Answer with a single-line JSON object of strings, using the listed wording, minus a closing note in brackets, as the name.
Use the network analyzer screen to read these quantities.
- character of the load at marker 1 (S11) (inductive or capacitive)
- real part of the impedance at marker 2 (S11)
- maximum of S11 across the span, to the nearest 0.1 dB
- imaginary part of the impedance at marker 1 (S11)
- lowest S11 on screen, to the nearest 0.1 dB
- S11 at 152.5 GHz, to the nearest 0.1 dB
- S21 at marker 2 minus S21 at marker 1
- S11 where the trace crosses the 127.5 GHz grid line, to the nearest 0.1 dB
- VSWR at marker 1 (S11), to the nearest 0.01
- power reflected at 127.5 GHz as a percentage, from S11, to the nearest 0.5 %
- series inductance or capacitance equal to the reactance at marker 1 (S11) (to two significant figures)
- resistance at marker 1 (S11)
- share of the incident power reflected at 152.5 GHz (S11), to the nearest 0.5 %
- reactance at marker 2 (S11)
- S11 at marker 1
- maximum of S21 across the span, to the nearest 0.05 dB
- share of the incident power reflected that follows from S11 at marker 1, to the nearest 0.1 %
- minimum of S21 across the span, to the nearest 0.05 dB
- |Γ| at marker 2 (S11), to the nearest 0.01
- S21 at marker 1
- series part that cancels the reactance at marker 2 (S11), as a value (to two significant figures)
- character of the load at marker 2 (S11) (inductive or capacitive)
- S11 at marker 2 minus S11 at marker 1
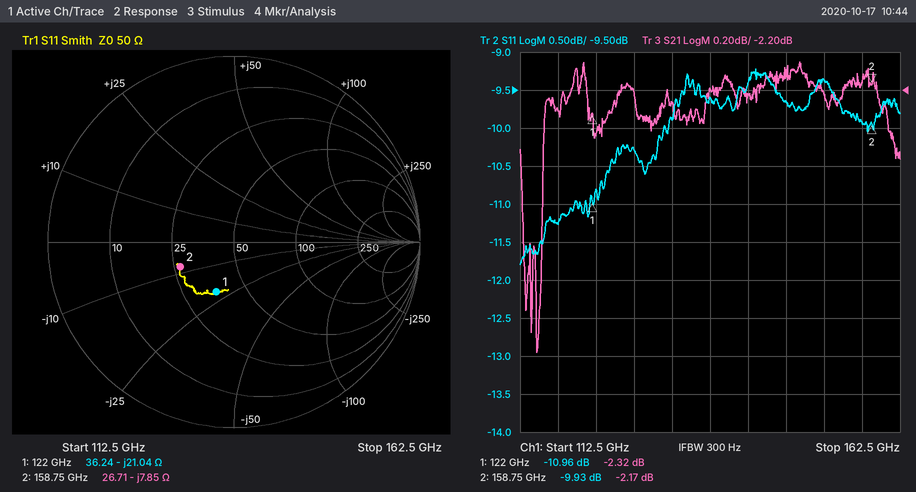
{"character of the load at marker 1 (S11)": "capacitive", "real part of the impedance at marker 2": "26.71 Ω", "maximum of S11 across the span, to the nearest 0.1 dB": "-9.2 dB", "imaginary part of the impedance at marker 1": "-21.04 Ω", "lowest S11 on screen, to the nearest 0.1 dB": "-11.8 dB", "S11 at 152.5 GHz, to the nearest 0.1 dB": "-9.4 dB", "S21 at marker 2 minus S21 at marker 1": "0.15 dB", "S11 where the trace crosses the 127.5 GHz grid line, to the nearest 0.1 dB": "-10.3 dB", "VSWR at marker 1 (S11), to the nearest 0.01": "1.79", "power reflected at 127.5 GHz as a percentage, from S11, to the nearest 0.5 %": "9.5 %", "series inductance or capacitance equal to the reactance at marker 1 (S11)": "62 fF", "resistance at marker 1": "36.24 Ω", "share of the incident power reflected at 152.5 GHz (S11), to the nearest 0.5 %": "11.5 %", "reactance at marker 2": "-7.85 Ω", "S11 at marker 1": "-10.96 dB", "maximum of S21 across the span, to the nearest 0.05 dB": "-2.05 dB", "share of the incident power reflected that follows from S11 at marker 1, to the nearest 0.1 %": "8.0 %", "minimum of S21 across the span, to the nearest 0.05 dB": "-3.60 dB", "|Γ| at marker 2 (S11), to the nearest 0.01": "0.32", "S21 at marker 1": "-2.32 dB", "series part that cancels the reactance at marker 2 (S11), as a value": "7.9 pH", "character of the load at marker 2 (S11)": "capacitive", "S11 at marker 2 minus S11 at marker 1": "1.03 dB"}
